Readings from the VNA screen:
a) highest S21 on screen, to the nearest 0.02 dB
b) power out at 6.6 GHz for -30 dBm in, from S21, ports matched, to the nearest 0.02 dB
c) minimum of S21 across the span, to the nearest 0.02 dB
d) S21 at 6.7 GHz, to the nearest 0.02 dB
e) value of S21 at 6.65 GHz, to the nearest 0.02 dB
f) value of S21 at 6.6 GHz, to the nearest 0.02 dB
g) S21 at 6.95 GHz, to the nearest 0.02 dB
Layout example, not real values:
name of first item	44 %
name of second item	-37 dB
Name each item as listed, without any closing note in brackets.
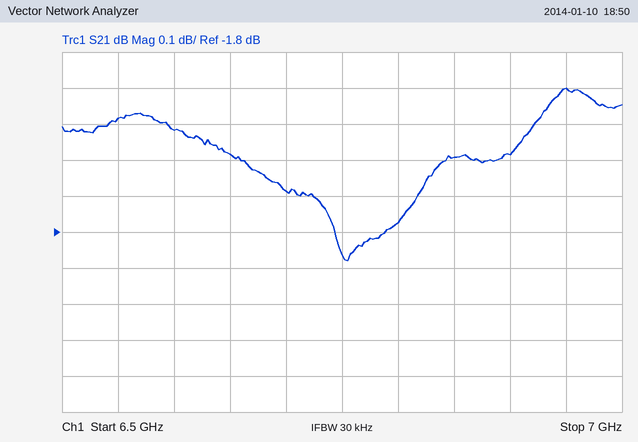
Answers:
highest S21 on screen, to the nearest 0.02 dB	-1.40 dB
power out at 6.6 GHz for -30 dBm in, from S21, ports matched, to the nearest 0.02 dB	-31.52 dBm
minimum of S21 across the span, to the nearest 0.02 dB	-1.88 dB
S21 at 6.7 GHz, to the nearest 0.02 dB	-1.68 dB
value of S21 at 6.65 GHz, to the nearest 0.02 dB	-1.58 dB
value of S21 at 6.6 GHz, to the nearest 0.02 dB	-1.52 dB
S21 at 6.95 GHz, to the nearest 0.02 dB	-1.40 dB
